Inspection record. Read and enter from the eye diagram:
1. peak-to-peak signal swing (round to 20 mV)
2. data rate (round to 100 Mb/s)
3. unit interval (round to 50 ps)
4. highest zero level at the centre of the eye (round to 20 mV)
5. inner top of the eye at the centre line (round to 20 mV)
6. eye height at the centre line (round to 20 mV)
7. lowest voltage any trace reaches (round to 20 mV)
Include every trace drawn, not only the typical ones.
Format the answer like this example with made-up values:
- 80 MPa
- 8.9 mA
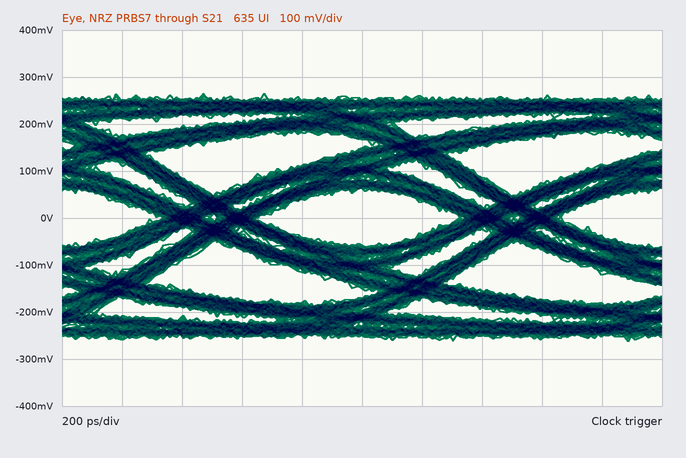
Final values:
- 520 mV
- 1.0 Gb/s
- 1.00 ns
- -60 mV
- 60 mV
- 120 mV
- -260 mV
